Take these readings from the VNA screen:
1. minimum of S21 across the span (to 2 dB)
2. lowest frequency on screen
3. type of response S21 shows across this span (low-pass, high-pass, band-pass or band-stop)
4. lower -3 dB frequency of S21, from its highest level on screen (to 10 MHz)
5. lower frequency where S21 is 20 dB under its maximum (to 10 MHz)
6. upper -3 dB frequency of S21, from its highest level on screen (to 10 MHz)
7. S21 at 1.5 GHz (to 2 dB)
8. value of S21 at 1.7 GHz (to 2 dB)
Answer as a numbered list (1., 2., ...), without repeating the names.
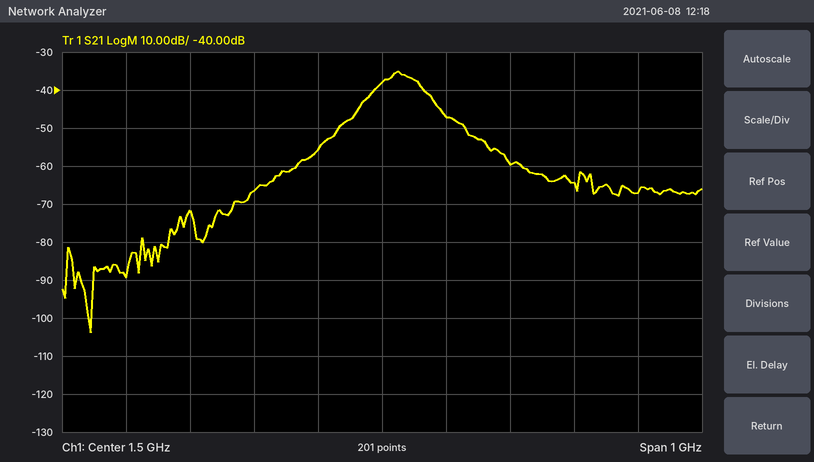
1. -104 dB
2. 1 GHz
3. band-pass
4. 1.50 GHz
5. 1.40 GHz
6. 1.56 GHz
7. -38 dB
8. -60 dB
